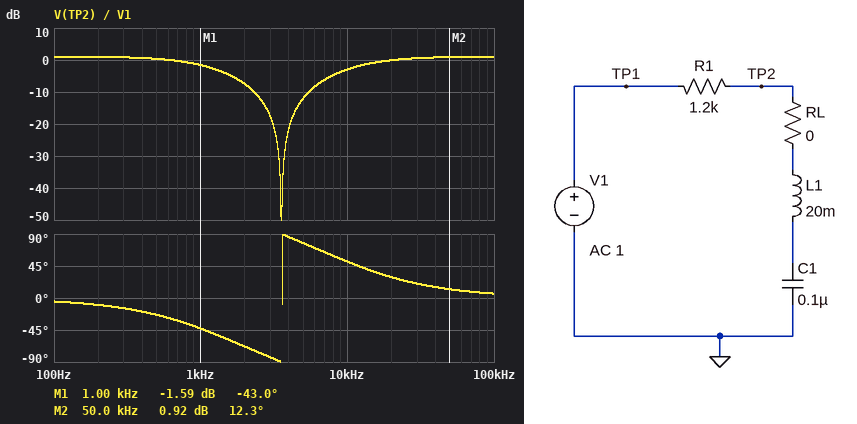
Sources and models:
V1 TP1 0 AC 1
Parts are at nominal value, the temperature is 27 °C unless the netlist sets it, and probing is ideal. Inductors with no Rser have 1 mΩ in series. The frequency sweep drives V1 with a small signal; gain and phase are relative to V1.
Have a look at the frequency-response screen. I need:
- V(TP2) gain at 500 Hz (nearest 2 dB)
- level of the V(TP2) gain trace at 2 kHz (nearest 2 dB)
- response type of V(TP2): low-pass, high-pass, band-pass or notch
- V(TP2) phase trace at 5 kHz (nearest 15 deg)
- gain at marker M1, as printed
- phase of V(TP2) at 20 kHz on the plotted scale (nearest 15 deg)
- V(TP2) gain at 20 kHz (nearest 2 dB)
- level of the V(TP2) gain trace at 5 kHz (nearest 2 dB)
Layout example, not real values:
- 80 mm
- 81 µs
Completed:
- 0 dB
- -8 dB
- notch
- 75 deg
- -1.59 dB
- 30 deg
- 0 dB
- -12 dB
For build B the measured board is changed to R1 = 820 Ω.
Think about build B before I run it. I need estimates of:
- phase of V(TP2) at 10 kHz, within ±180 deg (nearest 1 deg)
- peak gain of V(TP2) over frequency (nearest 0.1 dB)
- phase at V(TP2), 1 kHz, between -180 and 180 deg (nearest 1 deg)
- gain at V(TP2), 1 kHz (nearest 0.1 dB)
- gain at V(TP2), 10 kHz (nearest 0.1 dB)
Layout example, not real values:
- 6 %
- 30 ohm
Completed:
- 37 deg
- 0 dB
- -29 deg
- -1.2 dB
- -1.9 dB
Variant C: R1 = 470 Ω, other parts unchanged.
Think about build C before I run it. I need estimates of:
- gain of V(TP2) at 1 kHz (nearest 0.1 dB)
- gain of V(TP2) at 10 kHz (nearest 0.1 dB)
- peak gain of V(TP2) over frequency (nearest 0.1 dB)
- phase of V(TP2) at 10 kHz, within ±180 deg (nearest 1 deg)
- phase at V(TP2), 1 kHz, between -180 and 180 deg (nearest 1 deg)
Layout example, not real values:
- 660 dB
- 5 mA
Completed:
- 0.2 dB
- -0.1 dB
- 0.7 dB
- 25 deg
- -19 deg
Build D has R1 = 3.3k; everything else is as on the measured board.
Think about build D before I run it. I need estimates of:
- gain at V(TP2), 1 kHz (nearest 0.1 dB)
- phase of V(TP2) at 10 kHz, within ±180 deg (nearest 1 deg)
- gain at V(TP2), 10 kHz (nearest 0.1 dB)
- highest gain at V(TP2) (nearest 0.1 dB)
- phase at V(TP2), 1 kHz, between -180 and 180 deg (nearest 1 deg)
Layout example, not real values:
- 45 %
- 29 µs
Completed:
- -7.6 dB
- 75 deg
- -9.9 dB
- 1.9 dB
- -70 deg
